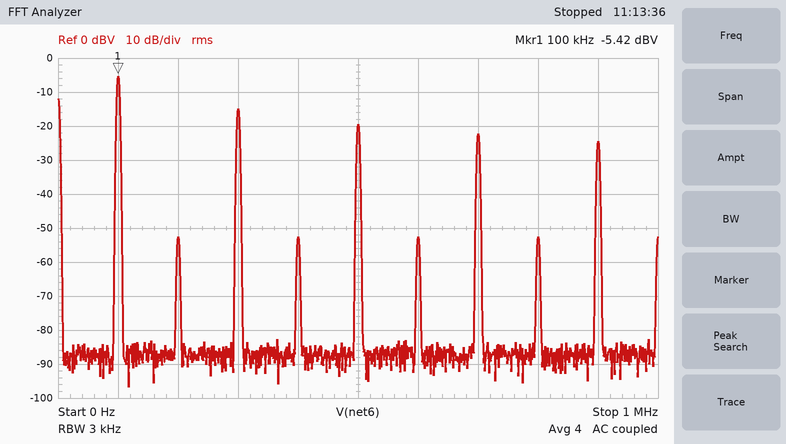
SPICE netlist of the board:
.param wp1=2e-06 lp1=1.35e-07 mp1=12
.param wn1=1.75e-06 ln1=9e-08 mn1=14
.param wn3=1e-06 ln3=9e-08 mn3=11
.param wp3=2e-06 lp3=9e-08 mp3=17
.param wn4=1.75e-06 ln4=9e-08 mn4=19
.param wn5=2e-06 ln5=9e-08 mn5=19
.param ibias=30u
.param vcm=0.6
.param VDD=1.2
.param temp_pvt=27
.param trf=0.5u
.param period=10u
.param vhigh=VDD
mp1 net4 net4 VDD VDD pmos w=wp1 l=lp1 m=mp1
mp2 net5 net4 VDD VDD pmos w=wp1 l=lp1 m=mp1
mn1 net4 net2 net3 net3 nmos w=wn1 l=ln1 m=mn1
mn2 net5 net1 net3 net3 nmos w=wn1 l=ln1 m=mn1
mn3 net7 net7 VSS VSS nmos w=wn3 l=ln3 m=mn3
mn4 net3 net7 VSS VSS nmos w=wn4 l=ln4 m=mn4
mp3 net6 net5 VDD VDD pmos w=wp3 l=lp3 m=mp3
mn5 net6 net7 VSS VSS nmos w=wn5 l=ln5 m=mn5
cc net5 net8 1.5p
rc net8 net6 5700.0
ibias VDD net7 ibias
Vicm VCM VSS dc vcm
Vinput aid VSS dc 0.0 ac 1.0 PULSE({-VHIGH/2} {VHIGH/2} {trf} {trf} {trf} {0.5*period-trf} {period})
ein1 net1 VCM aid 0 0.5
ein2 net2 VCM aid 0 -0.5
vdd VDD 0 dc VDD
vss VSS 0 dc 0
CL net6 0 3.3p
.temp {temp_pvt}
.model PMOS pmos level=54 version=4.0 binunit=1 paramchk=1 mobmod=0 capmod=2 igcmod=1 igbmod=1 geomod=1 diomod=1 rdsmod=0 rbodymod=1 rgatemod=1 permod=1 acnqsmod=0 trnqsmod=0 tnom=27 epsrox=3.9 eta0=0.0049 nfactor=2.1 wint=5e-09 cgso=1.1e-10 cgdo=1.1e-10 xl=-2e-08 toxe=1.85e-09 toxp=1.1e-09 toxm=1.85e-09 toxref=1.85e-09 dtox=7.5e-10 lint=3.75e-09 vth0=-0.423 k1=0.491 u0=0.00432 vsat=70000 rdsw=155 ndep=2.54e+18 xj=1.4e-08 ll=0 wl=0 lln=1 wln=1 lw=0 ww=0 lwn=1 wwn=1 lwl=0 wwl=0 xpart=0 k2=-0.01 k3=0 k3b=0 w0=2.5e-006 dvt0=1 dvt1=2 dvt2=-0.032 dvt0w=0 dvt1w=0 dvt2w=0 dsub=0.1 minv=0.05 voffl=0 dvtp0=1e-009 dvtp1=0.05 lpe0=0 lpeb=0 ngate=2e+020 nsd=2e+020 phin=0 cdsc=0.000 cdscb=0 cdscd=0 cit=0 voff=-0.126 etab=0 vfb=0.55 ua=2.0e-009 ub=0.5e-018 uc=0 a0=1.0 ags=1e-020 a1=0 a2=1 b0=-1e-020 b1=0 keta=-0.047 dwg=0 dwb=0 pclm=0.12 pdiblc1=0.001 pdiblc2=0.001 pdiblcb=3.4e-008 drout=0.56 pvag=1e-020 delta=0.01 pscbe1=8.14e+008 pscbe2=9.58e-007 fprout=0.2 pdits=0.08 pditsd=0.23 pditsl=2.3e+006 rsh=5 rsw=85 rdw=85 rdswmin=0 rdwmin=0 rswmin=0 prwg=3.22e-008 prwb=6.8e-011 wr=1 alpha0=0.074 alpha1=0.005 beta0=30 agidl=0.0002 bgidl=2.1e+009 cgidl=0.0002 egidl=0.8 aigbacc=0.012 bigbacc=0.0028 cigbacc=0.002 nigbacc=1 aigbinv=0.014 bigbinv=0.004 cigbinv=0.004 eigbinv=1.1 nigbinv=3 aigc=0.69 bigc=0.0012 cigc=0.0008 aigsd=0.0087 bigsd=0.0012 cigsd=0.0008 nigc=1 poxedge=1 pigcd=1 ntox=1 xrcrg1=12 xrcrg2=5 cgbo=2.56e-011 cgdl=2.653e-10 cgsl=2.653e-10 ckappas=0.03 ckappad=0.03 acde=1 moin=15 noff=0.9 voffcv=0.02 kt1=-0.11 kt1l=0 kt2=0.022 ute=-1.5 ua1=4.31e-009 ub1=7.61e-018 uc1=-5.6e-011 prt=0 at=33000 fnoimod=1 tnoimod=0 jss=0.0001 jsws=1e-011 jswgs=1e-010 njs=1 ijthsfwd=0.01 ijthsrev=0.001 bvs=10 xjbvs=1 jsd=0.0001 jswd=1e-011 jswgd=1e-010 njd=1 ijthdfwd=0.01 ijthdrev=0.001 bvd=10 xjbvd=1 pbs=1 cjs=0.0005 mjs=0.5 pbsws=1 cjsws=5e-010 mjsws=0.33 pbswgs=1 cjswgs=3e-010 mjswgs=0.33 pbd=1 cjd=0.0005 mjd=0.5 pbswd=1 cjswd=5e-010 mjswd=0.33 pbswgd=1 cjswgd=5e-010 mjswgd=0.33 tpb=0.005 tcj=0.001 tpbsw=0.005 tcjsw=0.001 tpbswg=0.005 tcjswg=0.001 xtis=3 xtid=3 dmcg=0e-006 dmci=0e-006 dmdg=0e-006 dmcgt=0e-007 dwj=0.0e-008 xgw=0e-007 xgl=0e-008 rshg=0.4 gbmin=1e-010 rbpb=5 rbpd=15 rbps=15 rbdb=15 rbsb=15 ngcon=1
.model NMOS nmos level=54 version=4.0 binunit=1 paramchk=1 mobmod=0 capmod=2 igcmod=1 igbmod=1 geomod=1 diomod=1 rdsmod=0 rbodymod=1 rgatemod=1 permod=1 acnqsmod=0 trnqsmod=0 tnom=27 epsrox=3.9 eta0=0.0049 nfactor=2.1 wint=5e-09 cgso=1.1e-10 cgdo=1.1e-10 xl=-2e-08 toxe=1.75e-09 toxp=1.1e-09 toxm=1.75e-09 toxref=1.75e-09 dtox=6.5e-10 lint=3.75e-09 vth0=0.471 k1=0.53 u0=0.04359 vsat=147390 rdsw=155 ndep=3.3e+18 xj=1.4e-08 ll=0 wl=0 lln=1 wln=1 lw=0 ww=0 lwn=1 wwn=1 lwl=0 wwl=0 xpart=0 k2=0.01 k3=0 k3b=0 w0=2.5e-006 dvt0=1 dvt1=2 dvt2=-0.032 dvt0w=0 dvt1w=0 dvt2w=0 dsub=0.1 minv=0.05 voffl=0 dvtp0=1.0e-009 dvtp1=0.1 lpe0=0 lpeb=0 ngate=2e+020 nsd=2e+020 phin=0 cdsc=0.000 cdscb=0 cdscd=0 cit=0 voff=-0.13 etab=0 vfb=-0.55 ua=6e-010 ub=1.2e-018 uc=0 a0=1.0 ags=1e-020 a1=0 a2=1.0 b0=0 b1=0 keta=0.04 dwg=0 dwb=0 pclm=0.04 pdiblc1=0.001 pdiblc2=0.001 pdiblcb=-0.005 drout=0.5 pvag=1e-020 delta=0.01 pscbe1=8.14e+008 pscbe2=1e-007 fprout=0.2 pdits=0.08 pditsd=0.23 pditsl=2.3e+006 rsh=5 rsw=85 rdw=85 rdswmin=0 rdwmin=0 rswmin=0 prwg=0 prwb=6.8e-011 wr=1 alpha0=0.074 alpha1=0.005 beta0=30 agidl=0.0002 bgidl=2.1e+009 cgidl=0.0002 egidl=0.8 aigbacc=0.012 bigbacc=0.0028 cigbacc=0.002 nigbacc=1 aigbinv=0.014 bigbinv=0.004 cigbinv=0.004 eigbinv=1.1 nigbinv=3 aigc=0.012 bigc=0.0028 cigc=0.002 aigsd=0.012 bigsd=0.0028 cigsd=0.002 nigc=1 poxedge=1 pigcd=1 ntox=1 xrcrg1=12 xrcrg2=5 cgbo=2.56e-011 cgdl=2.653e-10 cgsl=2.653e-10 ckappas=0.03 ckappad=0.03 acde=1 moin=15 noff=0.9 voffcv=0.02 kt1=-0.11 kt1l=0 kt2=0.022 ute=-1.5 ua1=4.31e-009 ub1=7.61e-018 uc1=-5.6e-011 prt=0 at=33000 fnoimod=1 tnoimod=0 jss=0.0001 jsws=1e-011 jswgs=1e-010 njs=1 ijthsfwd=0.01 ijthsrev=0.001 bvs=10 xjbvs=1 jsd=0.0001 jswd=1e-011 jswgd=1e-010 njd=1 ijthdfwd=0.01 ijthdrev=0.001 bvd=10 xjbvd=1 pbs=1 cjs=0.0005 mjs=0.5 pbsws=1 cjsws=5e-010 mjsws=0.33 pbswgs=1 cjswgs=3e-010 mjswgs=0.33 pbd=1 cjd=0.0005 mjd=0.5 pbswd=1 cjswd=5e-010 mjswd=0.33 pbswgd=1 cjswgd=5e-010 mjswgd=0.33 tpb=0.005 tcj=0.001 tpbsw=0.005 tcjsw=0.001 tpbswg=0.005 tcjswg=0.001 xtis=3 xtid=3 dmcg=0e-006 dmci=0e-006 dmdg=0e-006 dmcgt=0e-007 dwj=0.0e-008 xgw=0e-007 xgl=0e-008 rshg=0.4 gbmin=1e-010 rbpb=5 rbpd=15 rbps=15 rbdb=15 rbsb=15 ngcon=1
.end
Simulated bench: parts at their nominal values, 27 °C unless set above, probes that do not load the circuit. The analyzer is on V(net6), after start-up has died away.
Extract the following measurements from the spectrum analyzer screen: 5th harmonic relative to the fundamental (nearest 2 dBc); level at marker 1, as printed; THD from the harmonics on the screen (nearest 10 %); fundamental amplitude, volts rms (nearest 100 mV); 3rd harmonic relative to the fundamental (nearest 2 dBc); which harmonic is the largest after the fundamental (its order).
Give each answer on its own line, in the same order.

-14 dBc
-5.42 dBV
40 %
500 mV
-10 dBc
3
